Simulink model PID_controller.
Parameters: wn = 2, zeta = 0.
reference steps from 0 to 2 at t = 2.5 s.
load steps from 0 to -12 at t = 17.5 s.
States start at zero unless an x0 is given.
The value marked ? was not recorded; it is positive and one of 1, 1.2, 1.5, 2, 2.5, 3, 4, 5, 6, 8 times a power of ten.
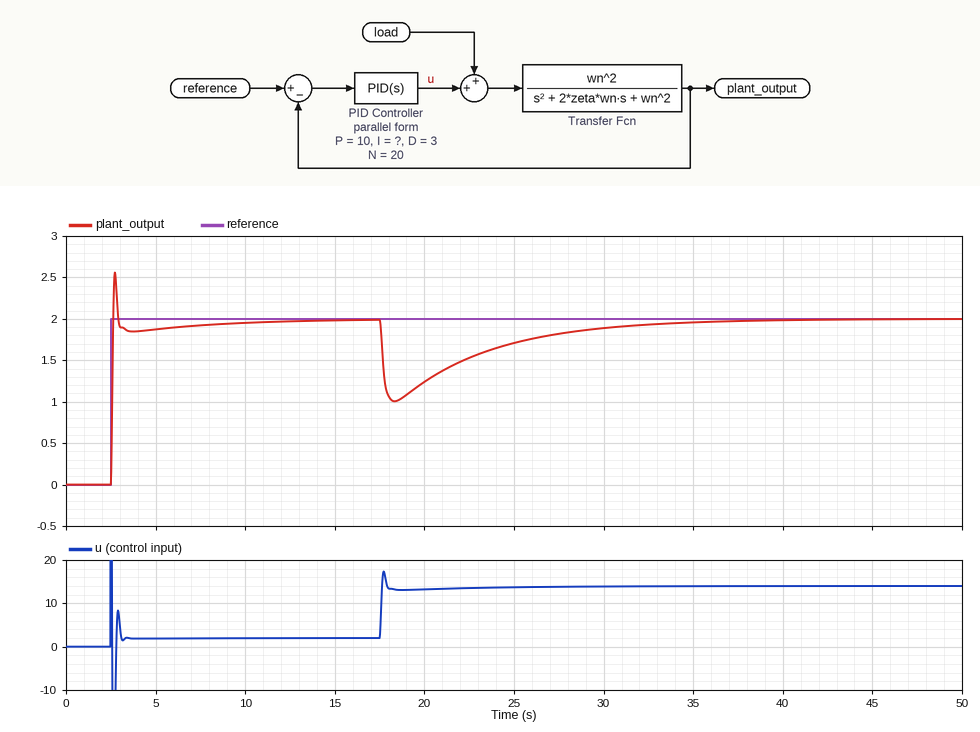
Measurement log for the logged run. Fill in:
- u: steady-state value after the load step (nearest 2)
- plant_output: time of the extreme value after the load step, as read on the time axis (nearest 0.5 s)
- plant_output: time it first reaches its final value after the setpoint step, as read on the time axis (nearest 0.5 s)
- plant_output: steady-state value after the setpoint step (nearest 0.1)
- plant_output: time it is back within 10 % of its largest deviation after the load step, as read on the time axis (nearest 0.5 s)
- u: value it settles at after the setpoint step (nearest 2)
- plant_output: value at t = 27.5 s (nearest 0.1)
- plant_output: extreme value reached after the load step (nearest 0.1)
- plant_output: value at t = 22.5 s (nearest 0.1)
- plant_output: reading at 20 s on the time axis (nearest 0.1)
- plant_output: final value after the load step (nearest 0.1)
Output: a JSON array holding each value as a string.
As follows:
["14", "18.5 s", "2.5 s", "2.0", "30.5 s", "2", "1.8", "1.0", "1.5", "1.2", "2.0"]
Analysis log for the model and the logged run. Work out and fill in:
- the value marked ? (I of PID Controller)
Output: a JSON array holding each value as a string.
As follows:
["2"]
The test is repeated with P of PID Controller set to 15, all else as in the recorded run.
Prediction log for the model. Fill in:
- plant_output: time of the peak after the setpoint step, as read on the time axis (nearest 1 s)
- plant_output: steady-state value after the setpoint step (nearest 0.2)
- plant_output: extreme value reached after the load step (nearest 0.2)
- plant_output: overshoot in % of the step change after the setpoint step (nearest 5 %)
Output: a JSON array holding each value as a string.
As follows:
["3 s", "2.0", "1.2", "35 %"]
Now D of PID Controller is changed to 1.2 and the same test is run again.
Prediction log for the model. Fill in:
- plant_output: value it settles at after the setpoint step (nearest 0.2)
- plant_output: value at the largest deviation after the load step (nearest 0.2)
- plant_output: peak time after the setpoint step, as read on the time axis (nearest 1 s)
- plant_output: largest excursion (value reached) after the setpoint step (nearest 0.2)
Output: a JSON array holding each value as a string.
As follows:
["2.0", "0.6", "3 s", "2.8"]
